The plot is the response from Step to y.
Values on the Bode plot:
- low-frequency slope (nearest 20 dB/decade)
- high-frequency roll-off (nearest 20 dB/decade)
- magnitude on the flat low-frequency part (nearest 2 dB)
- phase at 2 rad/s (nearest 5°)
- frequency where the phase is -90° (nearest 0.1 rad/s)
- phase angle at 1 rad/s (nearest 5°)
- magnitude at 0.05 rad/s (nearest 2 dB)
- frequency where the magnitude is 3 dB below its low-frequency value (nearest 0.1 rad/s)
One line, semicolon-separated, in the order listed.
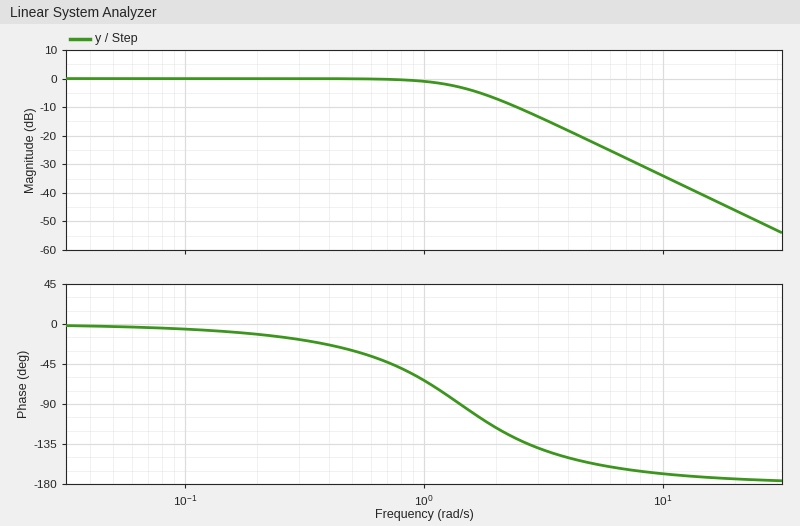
0 dB/decade; -40 dB/decade; 0 dB; -115°; 1.4 rad/s; -65°; 0 dB; 1.4 rad/s
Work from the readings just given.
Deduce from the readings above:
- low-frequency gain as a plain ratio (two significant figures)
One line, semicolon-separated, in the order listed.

1.0
